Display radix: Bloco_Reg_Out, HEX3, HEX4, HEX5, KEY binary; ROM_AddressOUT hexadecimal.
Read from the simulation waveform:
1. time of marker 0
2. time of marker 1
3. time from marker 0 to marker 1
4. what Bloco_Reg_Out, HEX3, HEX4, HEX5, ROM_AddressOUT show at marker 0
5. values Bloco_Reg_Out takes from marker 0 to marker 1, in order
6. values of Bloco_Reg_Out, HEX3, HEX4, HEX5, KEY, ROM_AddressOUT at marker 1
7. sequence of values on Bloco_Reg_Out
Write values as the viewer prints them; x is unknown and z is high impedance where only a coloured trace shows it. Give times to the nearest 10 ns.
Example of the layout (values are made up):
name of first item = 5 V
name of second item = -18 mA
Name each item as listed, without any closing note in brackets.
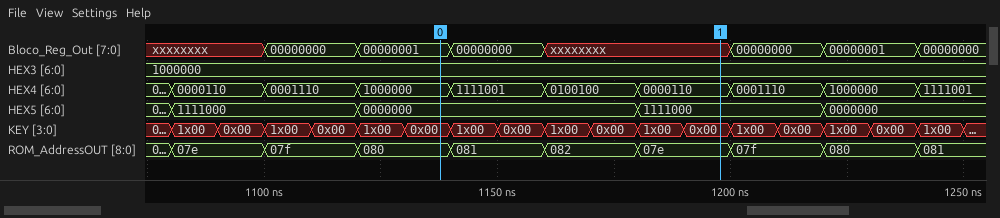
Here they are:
time of marker 0 = 1140 ns
time of marker 1 = 1200 ns
time from marker 0 to marker 1 = 60 ns
what Bloco_Reg_Out, HEX3, HEX4, HEX5, ROM_AddressOUT show at marker 0 = Bloco_Reg_Out=00000001, HEX3=1000000, HEX4=1000000, HEX5=0000000, ROM_AddressOUT=080
values Bloco_Reg_Out takes from marker 0 to marker 1, in order = 00000001, 00000000, xxxxxxxx
values of Bloco_Reg_Out, HEX3, HEX4, HEX5, KEY, ROM_AddressOUT at marker 1 = Bloco_Reg_Out=xxxxxxxx, HEX3=1000000, HEX4=0000110, HEX5=1111000, KEY=0x00, ROM_AddressOUT=07e
sequence of values on Bloco_Reg_Out = xxxxxxxx, 00000000, 00000001, 00000000, xxxxxxxx, 00000000, 00000001, 00000000
